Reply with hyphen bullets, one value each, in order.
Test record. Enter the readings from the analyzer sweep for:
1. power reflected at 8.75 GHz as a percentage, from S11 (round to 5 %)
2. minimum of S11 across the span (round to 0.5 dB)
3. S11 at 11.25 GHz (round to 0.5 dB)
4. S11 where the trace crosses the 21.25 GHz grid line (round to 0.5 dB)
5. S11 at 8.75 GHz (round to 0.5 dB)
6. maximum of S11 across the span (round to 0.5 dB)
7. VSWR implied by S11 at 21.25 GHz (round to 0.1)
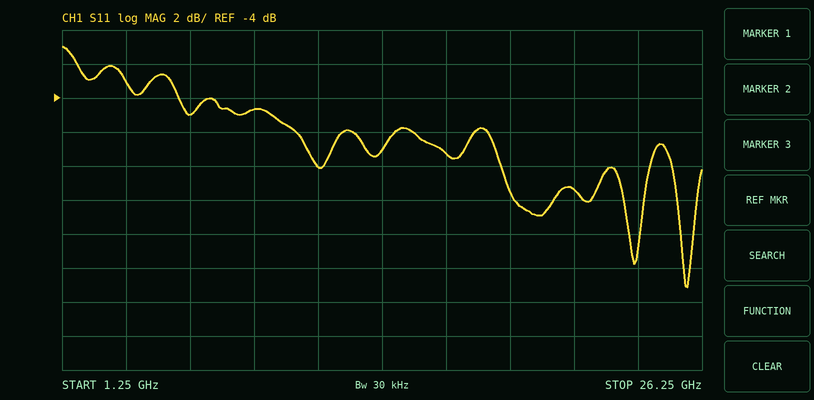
- 35 %
- -15.0 dB
- -8.0 dB
- -9.5 dB
- -4.5 dB
- -1.0 dB
- 2.0
